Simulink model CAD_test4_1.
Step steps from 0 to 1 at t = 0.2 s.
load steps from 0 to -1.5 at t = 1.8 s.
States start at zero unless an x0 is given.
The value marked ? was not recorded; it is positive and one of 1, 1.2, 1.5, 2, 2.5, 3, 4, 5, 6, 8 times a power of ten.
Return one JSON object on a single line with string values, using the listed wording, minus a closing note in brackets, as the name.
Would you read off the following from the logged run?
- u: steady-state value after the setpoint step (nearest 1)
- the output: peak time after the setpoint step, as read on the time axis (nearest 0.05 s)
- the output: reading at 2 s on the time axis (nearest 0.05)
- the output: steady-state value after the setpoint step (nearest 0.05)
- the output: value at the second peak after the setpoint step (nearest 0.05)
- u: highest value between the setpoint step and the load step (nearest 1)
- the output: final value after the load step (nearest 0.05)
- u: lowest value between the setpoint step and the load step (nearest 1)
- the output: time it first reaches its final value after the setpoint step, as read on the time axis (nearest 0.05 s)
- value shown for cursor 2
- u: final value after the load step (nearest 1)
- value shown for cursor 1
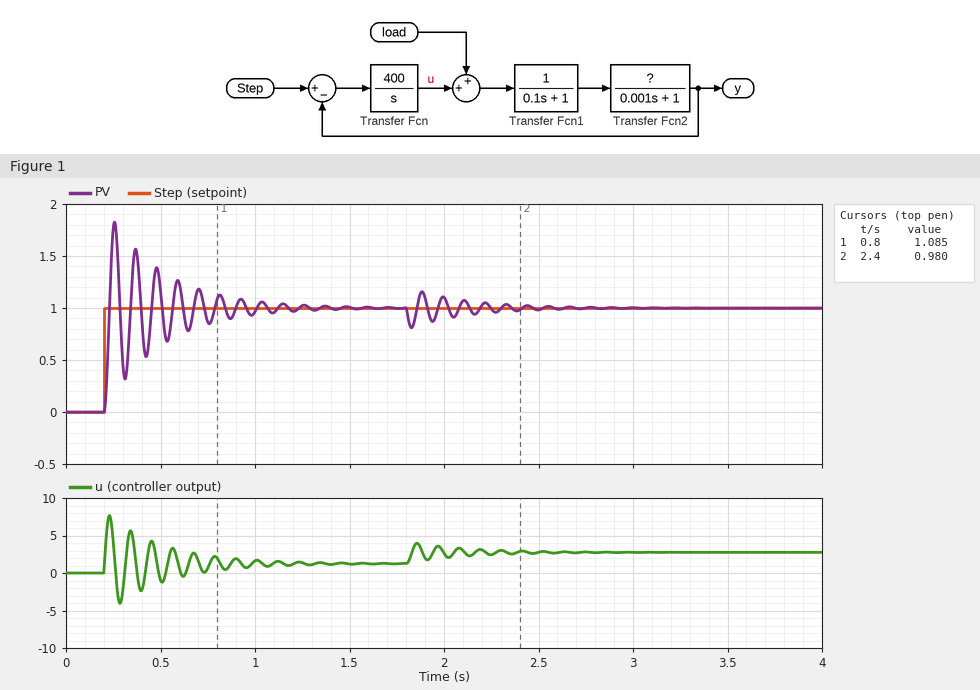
{"u: steady-state value after the setpoint step": "1", "the output: peak time after the setpoint step, as read on the time axis": "0.25 s", "the output: reading at 2 s on the time axis": "1.10", "the output: steady-state value after the setpoint step": "1.00", "the output: value at the second peak after the setpoint step": "1.55", "u: highest value between the setpoint step and the load step": "8", "the output: final value after the load step": "1.00", "u: lowest value between the setpoint step and the load step": "-4", "the output: time it first reaches its final value after the setpoint step, as read on the time axis": "0.25 s", "value shown for cursor 2": "0.980", "u: final value after the load step": "3", "value shown for cursor 1": "1.085"}
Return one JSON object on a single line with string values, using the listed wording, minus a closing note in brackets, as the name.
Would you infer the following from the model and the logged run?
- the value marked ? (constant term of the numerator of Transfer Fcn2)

{"the value marked ?": "0.8"}
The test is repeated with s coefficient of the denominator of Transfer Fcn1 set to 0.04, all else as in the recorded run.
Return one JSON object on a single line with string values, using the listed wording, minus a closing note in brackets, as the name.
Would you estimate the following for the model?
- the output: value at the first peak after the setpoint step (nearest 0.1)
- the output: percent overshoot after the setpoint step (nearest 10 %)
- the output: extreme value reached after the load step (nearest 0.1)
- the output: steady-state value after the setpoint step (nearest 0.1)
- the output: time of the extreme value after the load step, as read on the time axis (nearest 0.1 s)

{"the output: value at the first peak after the setpoint step": "1.7", "the output: percent overshoot after the setpoint step": "70 %", "the output: extreme value reached after the load step": "0.7", "the output: steady-state value after the setpoint step": "1.0", "the output: time of the extreme value after the load step, as read on the time axis": "1.8 s"}
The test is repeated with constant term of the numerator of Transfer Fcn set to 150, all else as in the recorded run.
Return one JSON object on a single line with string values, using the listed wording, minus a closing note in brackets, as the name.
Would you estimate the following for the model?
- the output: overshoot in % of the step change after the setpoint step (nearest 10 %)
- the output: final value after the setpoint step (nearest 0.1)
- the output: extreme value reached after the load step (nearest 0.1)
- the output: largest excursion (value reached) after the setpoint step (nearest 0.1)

{"the output: overshoot in % of the step change after the setpoint step": "70 %", "the output: final value after the setpoint step": "1.0", "the output: extreme value reached after the load step": "0.7", "the output: largest excursion (value reached) after the setpoint step": "1.7"}
